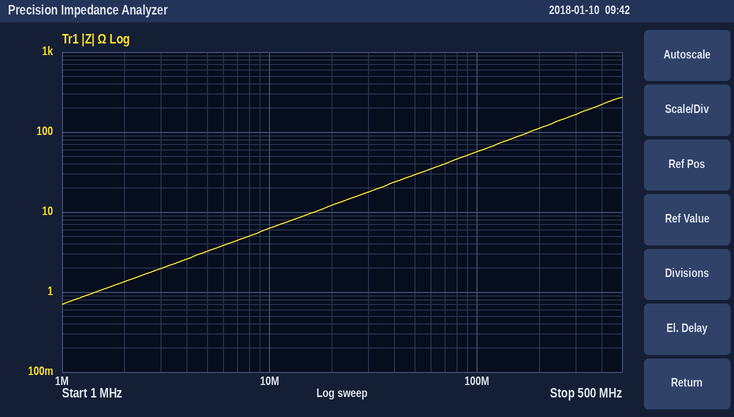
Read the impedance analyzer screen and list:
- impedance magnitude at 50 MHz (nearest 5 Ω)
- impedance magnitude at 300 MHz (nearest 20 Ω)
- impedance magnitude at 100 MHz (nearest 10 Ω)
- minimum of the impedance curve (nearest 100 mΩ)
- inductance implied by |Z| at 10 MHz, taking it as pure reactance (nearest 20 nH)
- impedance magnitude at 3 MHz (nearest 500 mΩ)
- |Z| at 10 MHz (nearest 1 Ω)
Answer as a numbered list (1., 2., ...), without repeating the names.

1. 30 Ω
2. 160 Ω
3. 60 Ω
4. 700 mΩ
5. 100 nH
6. 2.0 Ω
7. 6 Ω
